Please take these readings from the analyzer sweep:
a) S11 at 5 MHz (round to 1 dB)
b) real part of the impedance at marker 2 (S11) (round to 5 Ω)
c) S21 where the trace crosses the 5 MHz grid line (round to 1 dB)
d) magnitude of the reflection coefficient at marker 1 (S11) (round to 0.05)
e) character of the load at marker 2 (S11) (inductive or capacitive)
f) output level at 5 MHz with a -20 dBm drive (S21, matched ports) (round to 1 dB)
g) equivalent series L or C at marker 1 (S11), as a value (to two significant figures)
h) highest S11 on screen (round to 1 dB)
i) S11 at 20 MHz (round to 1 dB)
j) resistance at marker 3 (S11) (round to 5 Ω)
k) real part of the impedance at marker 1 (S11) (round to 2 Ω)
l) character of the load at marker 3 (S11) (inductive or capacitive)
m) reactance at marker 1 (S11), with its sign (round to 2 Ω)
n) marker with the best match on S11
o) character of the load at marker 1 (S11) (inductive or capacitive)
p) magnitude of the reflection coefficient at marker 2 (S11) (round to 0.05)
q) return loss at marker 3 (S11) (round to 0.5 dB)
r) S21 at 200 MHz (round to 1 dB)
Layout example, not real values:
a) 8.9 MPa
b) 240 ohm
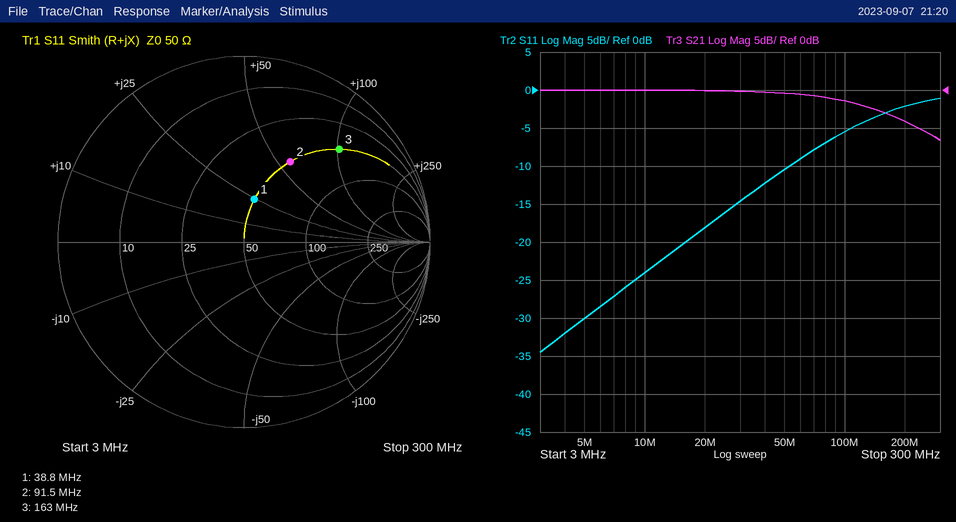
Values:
a) -30 dB
b) 50 Ω
c) 0 dB
d) 0.25
e) inductive
f) -20 dBm
g) 100 nH
h) -1 dB
i) -18 dB
j) 50 Ω
k) 50 Ω
l) inductive
m) +24 Ω
n) marker 1
o) inductive
p) 0.50
q) 3.0 dB
r) -4 dB
